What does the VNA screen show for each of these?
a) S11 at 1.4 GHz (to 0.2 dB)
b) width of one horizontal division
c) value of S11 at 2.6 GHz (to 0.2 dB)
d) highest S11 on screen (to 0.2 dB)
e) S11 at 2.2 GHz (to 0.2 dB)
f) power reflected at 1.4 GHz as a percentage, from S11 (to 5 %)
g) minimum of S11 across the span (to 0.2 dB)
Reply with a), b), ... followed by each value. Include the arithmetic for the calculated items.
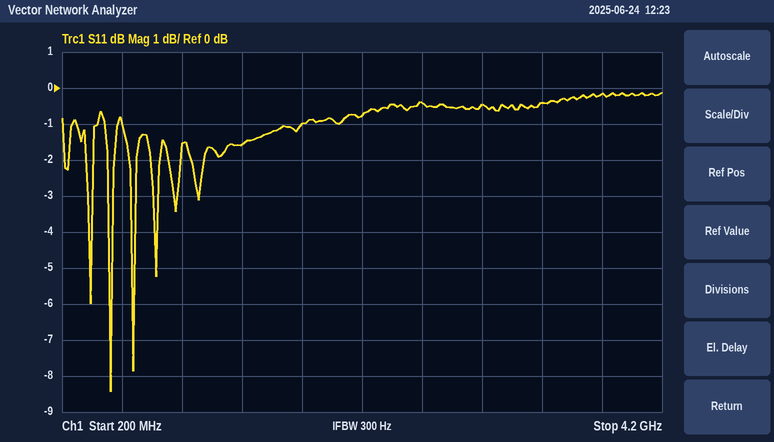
a) -1.6 dB
b) 400 MHz
c) -0.4 dB
d) -0.2 dB
e) -0.8 dB
f) 10^(-1.6/10) ≈ 69.2 %, so 70 % to the nearest 5 %
g) -8.4 dB
